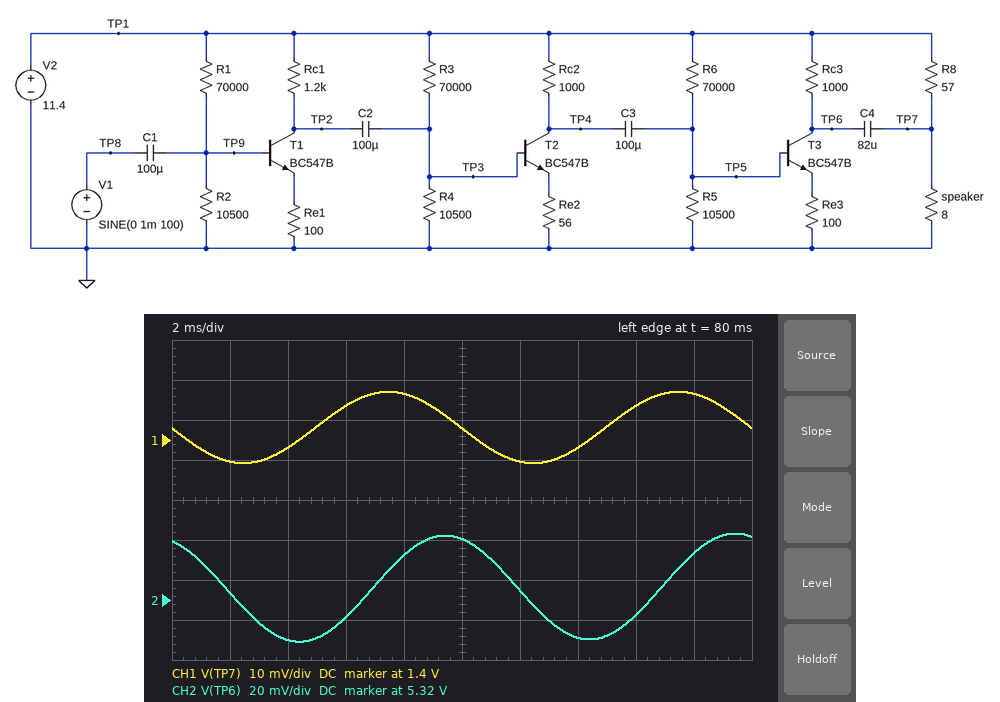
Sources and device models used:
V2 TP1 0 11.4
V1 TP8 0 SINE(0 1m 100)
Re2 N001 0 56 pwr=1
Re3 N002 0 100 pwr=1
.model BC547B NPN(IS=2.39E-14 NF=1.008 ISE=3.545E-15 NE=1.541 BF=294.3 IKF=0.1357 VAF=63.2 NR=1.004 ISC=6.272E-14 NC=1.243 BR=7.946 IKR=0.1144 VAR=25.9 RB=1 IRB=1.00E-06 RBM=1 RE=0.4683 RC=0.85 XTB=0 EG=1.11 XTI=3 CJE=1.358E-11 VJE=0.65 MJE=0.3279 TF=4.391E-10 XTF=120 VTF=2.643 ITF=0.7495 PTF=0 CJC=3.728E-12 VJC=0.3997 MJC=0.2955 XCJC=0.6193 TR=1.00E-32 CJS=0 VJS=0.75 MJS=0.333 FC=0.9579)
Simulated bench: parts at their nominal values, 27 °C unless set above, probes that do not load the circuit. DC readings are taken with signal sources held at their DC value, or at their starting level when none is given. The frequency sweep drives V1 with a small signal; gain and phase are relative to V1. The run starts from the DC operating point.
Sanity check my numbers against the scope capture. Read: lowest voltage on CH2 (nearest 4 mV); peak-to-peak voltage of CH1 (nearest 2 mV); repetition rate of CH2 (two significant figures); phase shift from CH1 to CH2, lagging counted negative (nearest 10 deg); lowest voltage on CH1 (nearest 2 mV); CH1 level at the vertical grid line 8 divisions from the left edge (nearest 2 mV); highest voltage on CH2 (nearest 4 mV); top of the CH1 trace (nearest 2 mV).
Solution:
5.300 V
18 mV
100 Hz
-70 deg
1.394 V
1.408 V
5.352 V
1.412 V
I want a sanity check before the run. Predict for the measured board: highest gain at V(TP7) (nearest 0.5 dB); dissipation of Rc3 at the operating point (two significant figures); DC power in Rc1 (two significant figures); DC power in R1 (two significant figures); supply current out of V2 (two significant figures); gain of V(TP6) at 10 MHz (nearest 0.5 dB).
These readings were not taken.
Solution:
19.0 dB
37 mW
44 mW
1.5 mW
200 mA
7.5 dB
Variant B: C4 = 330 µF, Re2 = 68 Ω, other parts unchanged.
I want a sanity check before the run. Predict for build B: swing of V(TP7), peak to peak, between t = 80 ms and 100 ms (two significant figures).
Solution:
15 mV
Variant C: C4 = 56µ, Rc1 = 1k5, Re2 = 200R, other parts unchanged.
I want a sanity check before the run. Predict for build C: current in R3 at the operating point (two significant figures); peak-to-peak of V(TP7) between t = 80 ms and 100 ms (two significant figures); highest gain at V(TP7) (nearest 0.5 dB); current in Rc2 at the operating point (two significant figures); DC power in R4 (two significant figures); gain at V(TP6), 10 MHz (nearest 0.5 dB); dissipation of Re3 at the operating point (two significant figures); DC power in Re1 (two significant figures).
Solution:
140 µA
6.6 mV
10.5 dB
3.5 mA
180 µW
4.5 dB
3.7 mW
3.6 mW
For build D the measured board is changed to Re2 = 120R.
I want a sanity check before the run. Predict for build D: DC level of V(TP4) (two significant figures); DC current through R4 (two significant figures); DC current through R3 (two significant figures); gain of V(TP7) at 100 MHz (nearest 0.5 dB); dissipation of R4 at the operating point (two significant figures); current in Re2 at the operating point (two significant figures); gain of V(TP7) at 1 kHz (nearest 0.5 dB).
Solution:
6.1 V
130 µA
140 µA
-19.5 dB
170 µW
5.3 mA
13.0 dB
